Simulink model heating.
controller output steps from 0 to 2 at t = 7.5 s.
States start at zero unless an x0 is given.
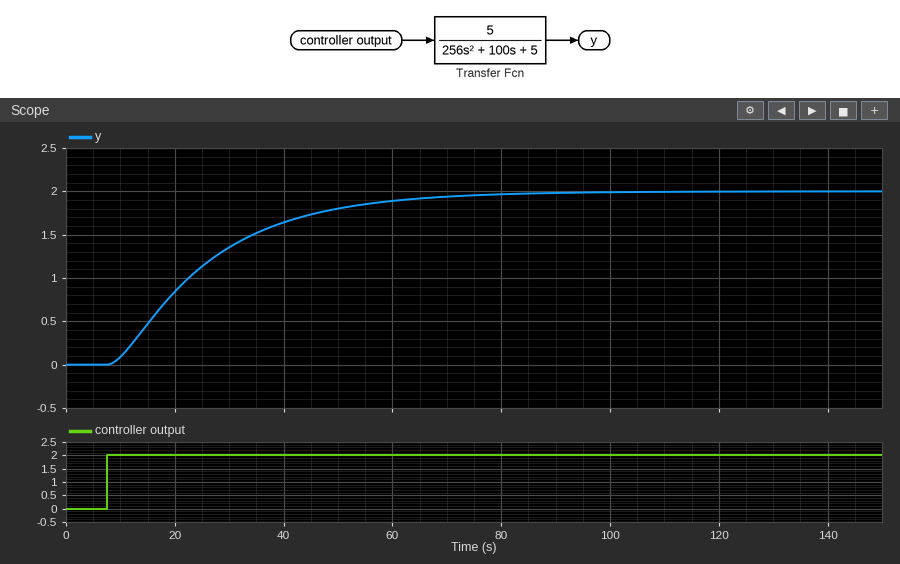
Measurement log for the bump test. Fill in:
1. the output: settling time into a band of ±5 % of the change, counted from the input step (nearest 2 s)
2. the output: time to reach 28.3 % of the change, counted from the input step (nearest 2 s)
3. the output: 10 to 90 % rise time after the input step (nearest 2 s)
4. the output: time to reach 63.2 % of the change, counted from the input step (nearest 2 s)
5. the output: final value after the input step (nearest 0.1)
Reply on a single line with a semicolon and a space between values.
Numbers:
54 s; 8 s; 38 s; 20 s; 2.0
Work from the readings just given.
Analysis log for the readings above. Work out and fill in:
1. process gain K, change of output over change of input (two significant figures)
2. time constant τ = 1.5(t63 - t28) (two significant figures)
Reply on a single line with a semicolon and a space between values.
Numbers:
1.0; 18 s
